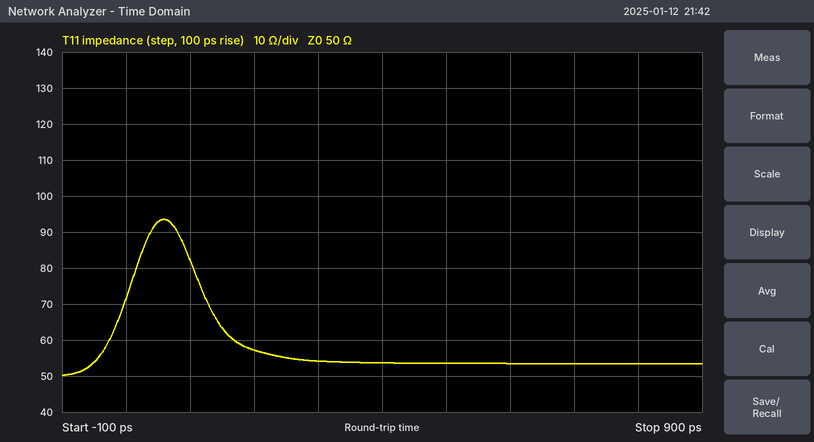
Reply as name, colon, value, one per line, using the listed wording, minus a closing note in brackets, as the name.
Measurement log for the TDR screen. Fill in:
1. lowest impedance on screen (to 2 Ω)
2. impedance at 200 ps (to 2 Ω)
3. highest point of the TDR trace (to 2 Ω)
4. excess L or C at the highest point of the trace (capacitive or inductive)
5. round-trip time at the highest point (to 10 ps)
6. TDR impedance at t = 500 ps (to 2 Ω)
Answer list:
lowest impedance on screen: 50 Ω
impedance at 200 ps: 58 Ω
highest point of the TDR trace: 94 Ω
excess L or C at the highest point of the trace: inductive
round-trip time at the highest point: 60 ps
TDR impedance at t = 500 ps: 54 Ω
